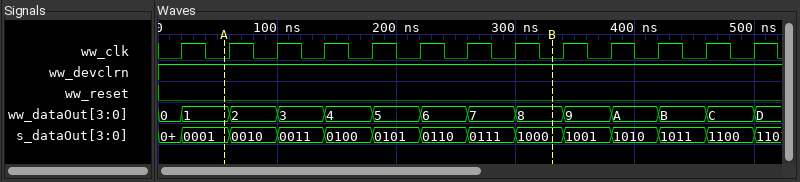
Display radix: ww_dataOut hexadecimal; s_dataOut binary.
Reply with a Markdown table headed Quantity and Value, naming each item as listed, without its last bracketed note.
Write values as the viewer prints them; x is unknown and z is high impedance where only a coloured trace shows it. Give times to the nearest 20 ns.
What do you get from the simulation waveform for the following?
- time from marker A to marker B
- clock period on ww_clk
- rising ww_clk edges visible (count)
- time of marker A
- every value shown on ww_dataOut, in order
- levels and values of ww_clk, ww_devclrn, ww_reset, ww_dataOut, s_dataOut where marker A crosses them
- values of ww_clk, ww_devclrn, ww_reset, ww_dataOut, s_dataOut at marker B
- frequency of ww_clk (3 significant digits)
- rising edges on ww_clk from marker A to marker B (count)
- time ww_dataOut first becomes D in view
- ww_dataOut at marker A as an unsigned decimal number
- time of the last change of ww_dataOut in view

| Quantity | Value |
|---|---|
| time from marker A to marker B | 280 ns |
| clock period on ww_clk | 40 ns |
| rising ww_clk edges visible | 13 |
| time of marker A | 60 ns |
| every value shown on ww_dataOut, in order | 0, 1, 2, 3, 4, 5, 6, 7, 8, 9, A, B, C, D |
| levels and values of ww_clk, ww_devclrn, ww_reset, ww_dataOut, s_dataOut where marker A crosses them | ww_clk=0, ww_devclrn=1, ww_reset=0, ww_dataOut=1, s_dataOut=0001 |
| values of ww_clk, ww_devclrn, ww_reset, ww_dataOut, s_dataOut at marker B | ww_clk=0, ww_devclrn=1, ww_reset=0, ww_dataOut=8, s_dataOut=1000 |
| frequency of ww_clk | 25.0 MHz |
| rising edges on ww_clk from marker A to marker B | 7 |
| time ww_dataOut first becomes D in view | 500 ns |
| ww_dataOut at marker A as an unsigned decimal number | 1 |
| time of the last change of ww_dataOut in view | 500 ns |
